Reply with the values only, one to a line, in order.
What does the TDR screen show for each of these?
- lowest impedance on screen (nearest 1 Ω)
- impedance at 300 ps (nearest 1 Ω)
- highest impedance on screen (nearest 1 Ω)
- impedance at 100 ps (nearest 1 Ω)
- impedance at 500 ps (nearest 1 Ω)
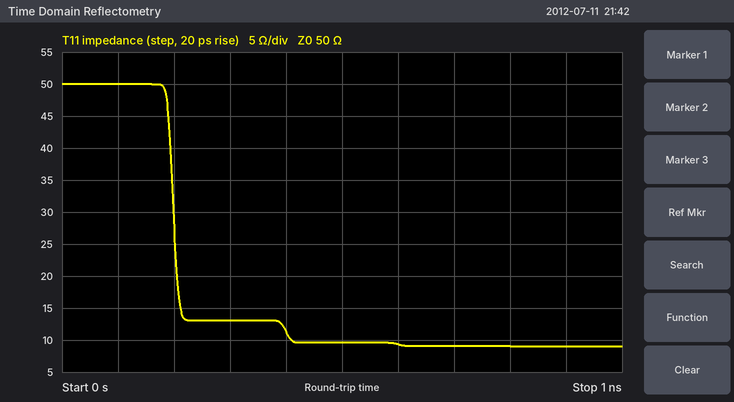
9 Ω
13 Ω
50 Ω
50 Ω
10 Ω
